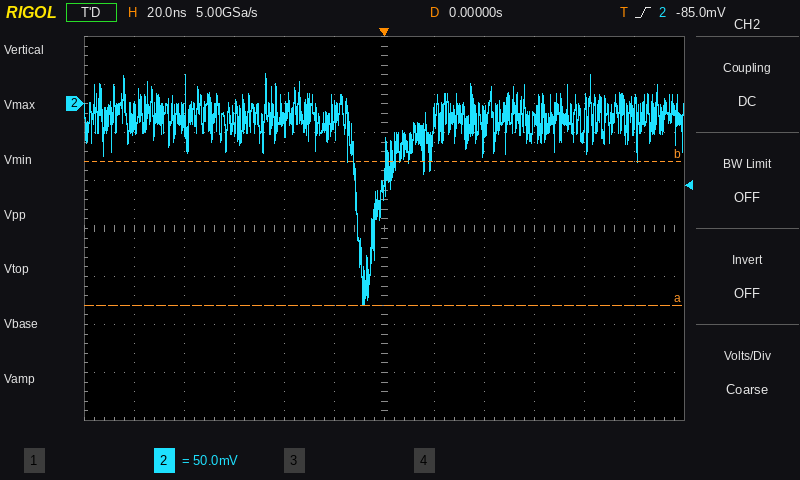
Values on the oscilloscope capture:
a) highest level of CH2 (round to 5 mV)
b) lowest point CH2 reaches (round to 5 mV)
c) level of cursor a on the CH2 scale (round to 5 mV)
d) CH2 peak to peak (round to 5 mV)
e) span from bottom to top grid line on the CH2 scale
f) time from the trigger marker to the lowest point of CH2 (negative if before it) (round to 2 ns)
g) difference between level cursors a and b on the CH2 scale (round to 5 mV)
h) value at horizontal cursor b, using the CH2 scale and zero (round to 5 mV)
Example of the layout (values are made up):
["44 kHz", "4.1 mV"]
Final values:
["30 mV", "-210 mV", "-210 mV", "240 mV", "400 mV", "-8 ns", "150 mV", "-60 mV"]
